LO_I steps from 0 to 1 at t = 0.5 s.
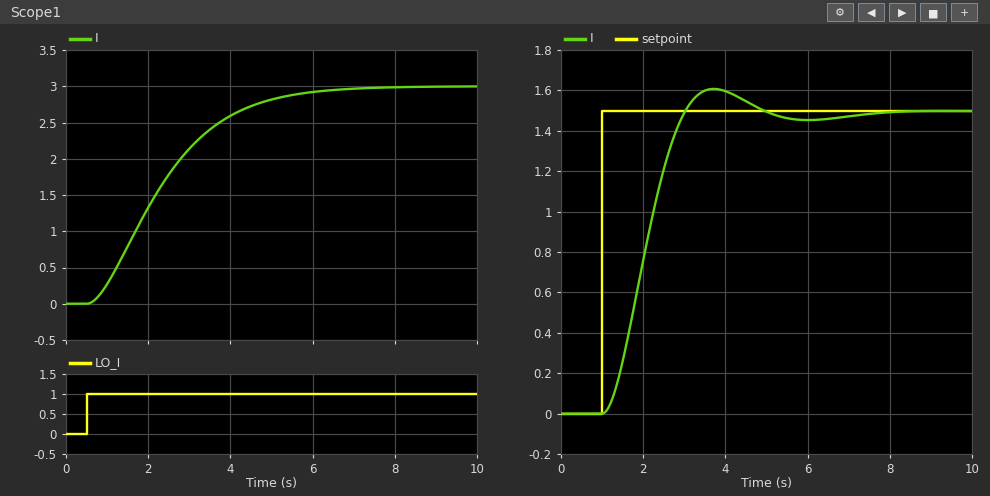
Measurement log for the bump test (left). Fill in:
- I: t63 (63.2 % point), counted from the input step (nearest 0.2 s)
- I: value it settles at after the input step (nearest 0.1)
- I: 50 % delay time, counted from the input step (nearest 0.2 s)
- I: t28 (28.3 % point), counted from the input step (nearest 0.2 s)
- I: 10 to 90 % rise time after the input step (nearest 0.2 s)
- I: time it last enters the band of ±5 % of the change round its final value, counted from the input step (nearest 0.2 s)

2.2 s
3.0
1.6 s
1.0 s
3.4 s
4.8 s
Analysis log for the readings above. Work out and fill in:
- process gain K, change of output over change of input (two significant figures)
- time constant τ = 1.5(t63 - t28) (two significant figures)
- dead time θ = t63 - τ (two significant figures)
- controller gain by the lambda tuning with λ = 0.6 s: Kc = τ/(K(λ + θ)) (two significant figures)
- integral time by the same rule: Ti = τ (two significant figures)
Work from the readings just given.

3.0
1.8 s
0.40 s
0.60
1.8 s
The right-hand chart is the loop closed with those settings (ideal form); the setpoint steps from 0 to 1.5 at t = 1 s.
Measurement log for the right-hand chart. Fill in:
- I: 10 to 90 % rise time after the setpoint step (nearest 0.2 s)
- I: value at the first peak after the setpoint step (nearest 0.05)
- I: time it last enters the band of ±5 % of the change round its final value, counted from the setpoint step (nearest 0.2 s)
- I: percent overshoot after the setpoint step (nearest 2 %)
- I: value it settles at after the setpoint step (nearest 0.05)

1.4 s
1.60
3.2 s
8 %
1.50
